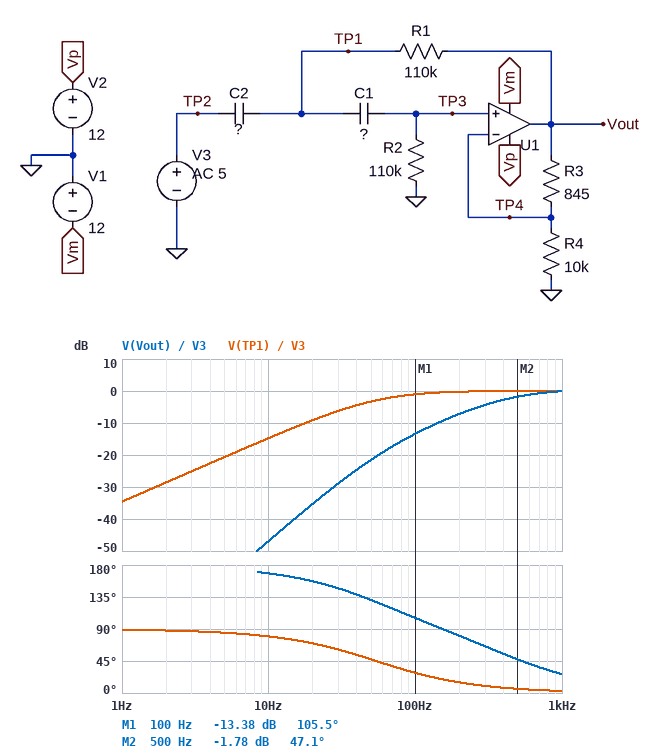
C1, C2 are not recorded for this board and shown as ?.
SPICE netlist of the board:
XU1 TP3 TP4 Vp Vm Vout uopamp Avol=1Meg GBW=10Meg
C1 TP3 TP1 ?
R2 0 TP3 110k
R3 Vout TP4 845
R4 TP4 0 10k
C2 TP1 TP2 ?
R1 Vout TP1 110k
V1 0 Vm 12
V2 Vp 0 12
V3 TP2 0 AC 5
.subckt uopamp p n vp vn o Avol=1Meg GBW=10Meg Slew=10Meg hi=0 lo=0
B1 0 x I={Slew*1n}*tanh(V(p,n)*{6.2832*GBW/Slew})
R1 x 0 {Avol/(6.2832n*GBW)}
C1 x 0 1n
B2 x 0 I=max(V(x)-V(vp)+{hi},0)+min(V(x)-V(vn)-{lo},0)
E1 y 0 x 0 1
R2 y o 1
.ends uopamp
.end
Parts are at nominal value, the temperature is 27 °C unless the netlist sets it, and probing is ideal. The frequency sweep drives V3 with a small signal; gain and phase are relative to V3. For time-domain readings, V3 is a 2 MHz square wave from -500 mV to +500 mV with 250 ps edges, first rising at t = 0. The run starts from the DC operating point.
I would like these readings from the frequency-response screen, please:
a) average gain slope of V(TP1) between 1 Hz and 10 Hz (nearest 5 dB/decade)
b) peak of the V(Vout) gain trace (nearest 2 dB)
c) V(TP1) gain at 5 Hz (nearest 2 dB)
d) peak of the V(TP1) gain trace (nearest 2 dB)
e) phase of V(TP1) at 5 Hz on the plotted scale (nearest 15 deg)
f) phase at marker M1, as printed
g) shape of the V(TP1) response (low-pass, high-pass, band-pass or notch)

20 dB/decade
0 dB
-20 dB
0 dB
90 deg
105.5 deg
high-pass
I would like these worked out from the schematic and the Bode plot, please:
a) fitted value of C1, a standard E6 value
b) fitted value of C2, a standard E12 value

3.3 nF
27 nF
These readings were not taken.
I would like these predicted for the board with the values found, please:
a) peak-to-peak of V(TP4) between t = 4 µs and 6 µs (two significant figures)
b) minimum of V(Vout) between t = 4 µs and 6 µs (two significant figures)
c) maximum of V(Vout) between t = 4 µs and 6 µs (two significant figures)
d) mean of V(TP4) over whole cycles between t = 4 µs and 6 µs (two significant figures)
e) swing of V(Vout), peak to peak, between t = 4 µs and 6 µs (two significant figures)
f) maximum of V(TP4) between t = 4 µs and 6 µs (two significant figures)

1.0 V
-9.9 mV
1.1 V
490 mV
1.1 V
990 mV
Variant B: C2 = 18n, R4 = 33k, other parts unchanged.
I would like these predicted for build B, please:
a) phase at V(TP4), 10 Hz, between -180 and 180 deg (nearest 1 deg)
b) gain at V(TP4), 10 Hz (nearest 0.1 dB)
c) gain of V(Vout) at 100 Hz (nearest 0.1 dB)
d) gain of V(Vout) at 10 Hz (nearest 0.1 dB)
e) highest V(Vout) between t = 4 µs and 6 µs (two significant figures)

172 deg
-51.0 dB
-15.0 dB
-50.8 dB
1.0 V
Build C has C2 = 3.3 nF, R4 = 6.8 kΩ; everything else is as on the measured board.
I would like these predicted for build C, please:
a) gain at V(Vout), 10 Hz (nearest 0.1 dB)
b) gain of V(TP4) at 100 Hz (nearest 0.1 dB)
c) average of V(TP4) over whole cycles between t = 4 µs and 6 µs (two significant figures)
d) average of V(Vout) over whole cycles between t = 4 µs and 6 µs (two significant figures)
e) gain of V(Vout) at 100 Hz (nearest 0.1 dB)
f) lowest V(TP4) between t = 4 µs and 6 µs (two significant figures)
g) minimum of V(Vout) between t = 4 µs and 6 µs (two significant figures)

-64.7 dB
-26.0 dB
490 mV
550 mV
-25.0 dB
-15 mV
-17 mV
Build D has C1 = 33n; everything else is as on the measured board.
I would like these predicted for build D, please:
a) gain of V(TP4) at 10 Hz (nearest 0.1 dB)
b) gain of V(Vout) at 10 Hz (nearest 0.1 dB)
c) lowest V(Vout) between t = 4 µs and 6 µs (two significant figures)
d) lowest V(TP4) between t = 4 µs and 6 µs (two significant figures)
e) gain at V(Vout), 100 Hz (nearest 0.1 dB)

-27.7 dB
-27.0 dB
-1.9 mV
-1.7 mV
-0.9 dB
